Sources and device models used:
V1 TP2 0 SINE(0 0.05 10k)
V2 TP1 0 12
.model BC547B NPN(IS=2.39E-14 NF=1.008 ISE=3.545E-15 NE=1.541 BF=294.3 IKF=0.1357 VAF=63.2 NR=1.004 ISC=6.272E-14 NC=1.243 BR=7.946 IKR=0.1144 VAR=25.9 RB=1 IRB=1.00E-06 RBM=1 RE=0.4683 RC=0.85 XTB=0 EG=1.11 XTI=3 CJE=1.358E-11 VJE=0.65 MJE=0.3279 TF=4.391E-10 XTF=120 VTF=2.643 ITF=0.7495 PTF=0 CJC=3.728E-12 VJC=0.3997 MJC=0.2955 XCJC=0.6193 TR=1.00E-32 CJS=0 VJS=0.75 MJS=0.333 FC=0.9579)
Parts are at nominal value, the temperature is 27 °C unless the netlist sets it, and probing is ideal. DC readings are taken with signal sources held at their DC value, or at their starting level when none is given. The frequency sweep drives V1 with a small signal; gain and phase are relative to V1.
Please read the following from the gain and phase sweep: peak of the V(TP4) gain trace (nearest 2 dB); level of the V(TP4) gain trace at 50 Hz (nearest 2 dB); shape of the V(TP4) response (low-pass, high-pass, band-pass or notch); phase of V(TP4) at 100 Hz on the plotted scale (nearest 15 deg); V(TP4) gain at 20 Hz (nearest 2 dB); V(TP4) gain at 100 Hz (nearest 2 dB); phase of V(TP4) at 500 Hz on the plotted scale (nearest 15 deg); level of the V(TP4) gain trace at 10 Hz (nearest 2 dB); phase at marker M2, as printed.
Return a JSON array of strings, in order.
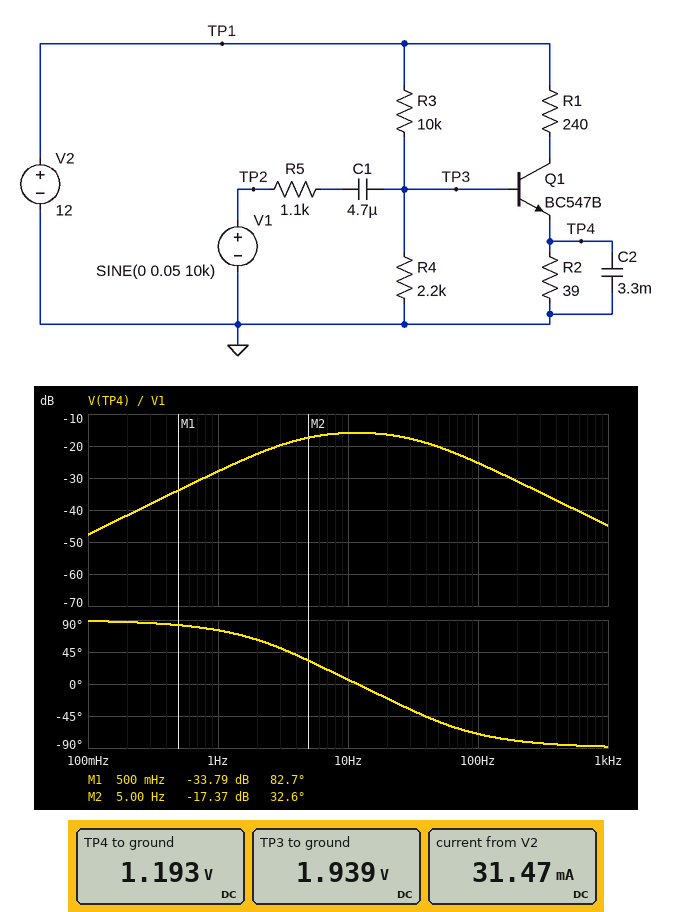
["-16 dB", "-20 dB", "band-pass", "-75 deg", "-16 dB", "-26 dB", "-90 deg", "-16 dB", "32.6 deg"]
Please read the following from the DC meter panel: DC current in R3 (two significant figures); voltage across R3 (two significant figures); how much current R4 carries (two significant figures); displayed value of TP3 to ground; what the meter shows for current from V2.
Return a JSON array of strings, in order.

["1.0 mA", "10 V", "880 µA", "1.939 V", "31.47 mA"]
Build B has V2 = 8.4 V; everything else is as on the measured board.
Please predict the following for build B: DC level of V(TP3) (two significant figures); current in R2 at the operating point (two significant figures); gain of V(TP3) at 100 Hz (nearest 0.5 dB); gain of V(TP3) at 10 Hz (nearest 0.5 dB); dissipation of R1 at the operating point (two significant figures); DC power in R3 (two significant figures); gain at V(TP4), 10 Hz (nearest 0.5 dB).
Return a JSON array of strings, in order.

["1.4 V", "17 mA", "-11.5 dB", "-14.0 dB", "71 mW", "4.9 mW", "-15.5 dB"]
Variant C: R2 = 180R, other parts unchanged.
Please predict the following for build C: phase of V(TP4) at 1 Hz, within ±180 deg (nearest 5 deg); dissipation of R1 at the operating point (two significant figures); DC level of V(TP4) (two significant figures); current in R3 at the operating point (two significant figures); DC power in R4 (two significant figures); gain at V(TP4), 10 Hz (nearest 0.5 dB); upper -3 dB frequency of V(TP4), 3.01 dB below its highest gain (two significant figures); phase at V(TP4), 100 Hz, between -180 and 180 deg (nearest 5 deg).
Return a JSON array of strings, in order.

["75 deg", "15 mW", "1.4 V", "990 µA", "2.0 mW", "-15.0 dB", "30 Hz", "-75 deg"]
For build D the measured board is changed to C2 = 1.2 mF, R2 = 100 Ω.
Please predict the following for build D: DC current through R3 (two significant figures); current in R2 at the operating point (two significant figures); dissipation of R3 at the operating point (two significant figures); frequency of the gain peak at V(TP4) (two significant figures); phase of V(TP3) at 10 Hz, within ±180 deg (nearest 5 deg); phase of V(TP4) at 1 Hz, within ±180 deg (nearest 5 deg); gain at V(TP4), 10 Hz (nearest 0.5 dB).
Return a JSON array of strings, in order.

["990 µA", "14 mA", "9.8 mW", "18 Hz", "35 deg", "80 deg", "-10.5 dB"]
